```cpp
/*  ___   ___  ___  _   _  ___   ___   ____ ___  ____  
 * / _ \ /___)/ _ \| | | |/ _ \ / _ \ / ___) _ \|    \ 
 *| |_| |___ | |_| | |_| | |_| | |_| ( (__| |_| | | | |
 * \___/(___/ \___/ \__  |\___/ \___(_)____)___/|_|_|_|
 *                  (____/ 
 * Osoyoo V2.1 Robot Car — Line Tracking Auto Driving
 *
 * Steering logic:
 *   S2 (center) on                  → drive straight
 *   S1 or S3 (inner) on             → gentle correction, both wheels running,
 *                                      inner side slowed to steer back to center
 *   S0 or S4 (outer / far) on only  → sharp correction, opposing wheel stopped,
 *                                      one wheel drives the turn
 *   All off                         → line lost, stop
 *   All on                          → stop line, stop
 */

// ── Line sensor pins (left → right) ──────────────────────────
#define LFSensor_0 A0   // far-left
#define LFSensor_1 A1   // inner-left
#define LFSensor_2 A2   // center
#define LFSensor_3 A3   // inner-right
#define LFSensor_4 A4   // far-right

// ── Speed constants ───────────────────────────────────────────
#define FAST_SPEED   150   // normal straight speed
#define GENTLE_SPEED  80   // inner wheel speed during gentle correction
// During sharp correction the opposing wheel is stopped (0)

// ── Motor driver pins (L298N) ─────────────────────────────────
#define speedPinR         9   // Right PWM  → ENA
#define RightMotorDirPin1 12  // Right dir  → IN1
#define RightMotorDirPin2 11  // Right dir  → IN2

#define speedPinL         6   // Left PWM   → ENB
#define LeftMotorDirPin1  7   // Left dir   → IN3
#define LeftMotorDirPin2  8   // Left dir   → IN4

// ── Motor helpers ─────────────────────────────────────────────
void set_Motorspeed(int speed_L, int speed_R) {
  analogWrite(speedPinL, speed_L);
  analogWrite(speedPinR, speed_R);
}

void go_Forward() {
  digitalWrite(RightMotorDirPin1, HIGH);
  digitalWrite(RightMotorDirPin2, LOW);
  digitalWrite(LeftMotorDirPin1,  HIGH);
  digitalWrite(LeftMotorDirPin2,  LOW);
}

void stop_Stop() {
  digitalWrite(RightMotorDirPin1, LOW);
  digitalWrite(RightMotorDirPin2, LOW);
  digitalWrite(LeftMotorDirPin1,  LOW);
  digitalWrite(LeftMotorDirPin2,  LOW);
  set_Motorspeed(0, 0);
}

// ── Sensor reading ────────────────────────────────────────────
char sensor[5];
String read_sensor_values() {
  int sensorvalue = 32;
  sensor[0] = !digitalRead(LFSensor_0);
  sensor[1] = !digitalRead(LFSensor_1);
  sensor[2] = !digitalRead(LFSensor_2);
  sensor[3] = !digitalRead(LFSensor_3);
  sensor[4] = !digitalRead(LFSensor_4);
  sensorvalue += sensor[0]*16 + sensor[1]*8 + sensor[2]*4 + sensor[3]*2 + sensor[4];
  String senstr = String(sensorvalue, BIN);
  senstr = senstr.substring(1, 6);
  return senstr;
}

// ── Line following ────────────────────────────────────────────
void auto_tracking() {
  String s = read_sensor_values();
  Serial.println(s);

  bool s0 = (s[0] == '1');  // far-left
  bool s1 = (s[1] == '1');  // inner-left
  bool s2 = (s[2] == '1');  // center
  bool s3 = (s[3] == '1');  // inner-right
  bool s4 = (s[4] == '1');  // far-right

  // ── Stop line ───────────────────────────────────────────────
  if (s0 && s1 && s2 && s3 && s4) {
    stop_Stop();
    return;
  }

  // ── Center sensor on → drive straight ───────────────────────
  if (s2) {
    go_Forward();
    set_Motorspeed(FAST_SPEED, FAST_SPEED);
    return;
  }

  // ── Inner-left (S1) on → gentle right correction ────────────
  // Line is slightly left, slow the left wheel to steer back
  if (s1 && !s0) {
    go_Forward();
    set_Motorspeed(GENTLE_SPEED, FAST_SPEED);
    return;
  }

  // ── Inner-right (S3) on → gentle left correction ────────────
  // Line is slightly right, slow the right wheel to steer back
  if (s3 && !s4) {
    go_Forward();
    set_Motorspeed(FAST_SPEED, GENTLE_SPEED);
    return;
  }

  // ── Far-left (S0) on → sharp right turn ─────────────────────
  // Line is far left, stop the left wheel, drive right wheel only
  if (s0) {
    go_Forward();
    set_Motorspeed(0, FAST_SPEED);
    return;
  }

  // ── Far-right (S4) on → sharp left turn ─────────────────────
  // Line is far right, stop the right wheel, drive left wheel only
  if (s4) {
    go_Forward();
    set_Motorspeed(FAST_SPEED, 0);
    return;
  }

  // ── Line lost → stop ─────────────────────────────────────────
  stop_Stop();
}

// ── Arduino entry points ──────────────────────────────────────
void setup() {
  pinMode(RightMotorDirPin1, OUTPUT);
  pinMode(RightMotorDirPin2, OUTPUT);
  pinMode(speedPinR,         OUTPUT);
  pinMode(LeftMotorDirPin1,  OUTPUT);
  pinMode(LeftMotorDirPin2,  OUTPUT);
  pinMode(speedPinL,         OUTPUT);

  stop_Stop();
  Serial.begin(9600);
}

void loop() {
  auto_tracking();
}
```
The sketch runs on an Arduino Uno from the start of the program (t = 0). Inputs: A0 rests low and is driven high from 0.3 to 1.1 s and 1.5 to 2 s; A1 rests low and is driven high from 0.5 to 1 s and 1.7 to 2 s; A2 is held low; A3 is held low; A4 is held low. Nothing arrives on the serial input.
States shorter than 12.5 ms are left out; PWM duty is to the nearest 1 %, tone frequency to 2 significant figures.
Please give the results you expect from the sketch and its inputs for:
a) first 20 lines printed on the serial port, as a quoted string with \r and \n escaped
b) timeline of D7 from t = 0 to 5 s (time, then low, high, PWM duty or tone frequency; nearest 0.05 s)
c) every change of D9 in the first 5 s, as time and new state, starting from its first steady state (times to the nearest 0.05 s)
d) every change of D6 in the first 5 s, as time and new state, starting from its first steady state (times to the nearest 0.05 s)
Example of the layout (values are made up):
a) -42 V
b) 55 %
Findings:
a) "11111\r\n11111\r\n11111\r\n11111\r\n11111\r\n11111\r\n11111\r\n11111\r\n11111\r\n11111\r\n11111\r\n11111\r\n11111\r\n11111\r\n11111\r\n11111\r\n11111\r\n11111\r\n11111\r\n11111\r\n"
b) 0 s low; 0.3 s high; 1.1 s low; 1.5 s high; 2 s low
c) 0 s low; 0.3 s PWM 59 %; 1.1 s low; 1.5 s PWM 59 %; 2 s low
d) 0 s low; 0.3 s PWM 59 %; 1.1 s low; 1.5 s PWM 59 %; 2 s low
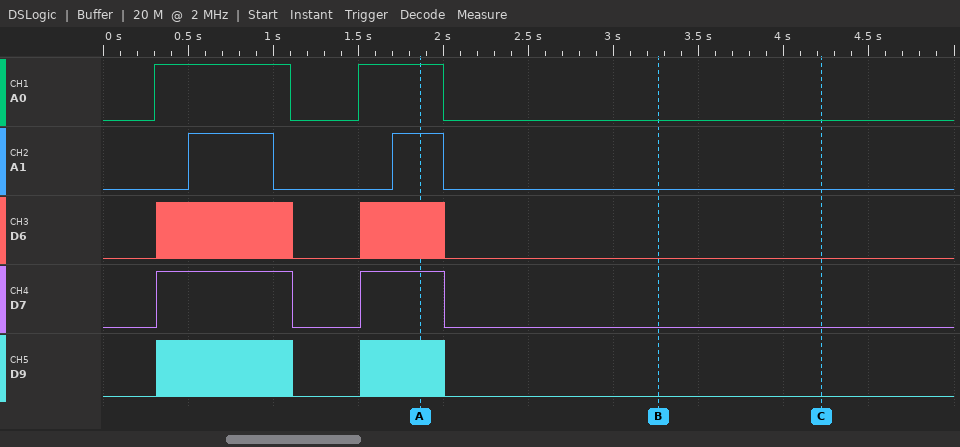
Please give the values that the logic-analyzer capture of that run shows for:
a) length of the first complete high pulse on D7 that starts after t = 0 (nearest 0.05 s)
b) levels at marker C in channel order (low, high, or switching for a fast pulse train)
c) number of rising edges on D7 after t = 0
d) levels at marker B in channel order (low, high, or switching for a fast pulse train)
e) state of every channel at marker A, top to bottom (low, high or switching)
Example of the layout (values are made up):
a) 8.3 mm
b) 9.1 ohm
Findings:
a) 0.80 s
b) A0 low, A1 low, D6 low, D7 low, D9 low
c) 2
d) A0 low, A1 low, D6 low, D7 low, D9 low
e) A0 high, A1 high, D6 switching, D7 high, D9 switching
